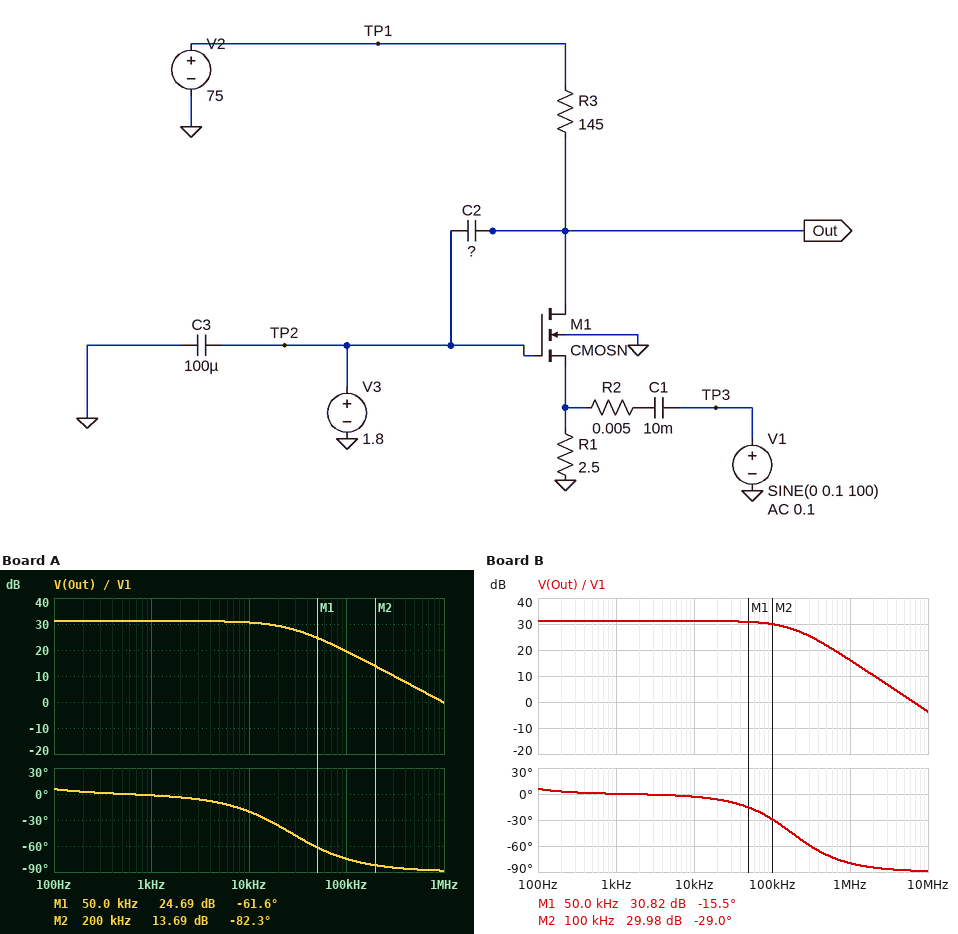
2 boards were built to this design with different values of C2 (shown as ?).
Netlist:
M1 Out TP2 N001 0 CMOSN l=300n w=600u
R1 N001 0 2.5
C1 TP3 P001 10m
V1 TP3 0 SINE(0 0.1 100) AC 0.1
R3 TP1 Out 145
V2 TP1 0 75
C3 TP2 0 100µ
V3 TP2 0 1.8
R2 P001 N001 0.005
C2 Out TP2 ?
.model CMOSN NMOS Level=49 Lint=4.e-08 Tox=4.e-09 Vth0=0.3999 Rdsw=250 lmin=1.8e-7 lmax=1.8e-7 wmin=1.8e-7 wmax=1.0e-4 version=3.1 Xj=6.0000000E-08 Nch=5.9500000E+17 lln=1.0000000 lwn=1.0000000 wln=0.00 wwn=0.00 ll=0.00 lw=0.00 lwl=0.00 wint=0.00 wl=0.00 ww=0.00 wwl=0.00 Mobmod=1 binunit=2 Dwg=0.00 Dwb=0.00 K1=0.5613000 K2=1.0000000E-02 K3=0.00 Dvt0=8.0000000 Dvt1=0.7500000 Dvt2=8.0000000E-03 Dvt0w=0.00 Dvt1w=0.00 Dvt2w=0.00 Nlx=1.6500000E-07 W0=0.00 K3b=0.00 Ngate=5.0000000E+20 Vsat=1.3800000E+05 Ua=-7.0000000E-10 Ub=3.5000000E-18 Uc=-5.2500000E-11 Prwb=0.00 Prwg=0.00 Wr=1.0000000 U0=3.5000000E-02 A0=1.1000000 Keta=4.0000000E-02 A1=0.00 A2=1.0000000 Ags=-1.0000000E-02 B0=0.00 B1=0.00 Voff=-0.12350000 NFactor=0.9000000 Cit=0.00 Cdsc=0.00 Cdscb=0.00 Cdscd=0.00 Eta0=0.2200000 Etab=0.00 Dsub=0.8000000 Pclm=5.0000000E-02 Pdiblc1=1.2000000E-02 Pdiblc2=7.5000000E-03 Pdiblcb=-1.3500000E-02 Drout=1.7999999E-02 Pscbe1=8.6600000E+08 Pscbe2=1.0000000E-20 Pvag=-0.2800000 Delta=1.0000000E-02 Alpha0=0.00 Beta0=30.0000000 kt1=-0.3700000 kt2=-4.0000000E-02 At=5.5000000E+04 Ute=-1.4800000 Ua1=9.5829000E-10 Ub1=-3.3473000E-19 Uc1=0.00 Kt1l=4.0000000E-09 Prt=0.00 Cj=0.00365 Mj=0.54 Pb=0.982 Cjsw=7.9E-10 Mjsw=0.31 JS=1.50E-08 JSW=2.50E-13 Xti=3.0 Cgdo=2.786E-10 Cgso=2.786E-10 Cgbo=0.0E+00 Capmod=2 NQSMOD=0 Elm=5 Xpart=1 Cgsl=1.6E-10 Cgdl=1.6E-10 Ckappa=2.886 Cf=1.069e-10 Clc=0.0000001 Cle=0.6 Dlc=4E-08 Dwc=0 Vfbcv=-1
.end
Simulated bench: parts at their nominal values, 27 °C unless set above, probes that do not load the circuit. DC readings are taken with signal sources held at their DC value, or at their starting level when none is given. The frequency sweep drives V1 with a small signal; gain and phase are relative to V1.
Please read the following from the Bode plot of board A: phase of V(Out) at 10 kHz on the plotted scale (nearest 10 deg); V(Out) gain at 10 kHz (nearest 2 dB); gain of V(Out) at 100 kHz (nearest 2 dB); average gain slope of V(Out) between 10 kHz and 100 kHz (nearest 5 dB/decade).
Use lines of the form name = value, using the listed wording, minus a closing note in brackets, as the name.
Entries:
phase of V(Out) at 10 kHz on the plotted scale = -20 deg
V(Out) gain at 10 kHz = 30 dB
gain of V(Out) at 100 kHz = 20 dB
average gain slope of V(Out) between 10 kHz and 100 kHz = -10 dB/decade
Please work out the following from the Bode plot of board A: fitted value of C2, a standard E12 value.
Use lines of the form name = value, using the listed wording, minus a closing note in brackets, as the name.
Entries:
fitted value of C2, a standard E12 value = 100 nF
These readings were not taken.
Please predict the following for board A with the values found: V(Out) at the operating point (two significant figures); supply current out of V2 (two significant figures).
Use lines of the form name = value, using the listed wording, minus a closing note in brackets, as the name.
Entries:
V(Out) at the operating point = 34 V
supply current out of V2 = 280 mA
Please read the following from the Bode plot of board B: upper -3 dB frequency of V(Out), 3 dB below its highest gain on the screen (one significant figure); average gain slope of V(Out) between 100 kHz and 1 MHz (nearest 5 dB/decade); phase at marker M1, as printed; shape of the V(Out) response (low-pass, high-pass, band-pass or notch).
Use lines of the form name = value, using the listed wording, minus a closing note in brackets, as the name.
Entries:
upper -3 dB frequency of V(Out), 3 dB below its highest gain on the screen = 200 kHz
average gain slope of V(Out) between 100 kHz and 1 MHz = -15 dB/decade
phase at marker M1, as printed = -15.5 deg
shape of the V(Out) response = low-pass
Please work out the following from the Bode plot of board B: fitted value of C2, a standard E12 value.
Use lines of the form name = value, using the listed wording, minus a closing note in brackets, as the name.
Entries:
fitted value of C2, a standard E12 value = 15 nF
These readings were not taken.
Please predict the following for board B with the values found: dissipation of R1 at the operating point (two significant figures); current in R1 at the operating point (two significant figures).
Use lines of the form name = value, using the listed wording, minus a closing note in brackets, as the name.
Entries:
dissipation of R1 at the operating point = 200 mW
current in R1 at the operating point = 280 mA
